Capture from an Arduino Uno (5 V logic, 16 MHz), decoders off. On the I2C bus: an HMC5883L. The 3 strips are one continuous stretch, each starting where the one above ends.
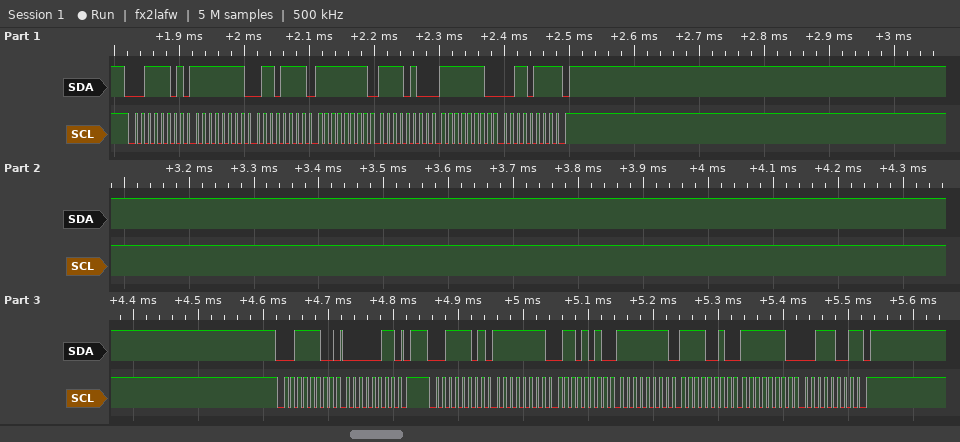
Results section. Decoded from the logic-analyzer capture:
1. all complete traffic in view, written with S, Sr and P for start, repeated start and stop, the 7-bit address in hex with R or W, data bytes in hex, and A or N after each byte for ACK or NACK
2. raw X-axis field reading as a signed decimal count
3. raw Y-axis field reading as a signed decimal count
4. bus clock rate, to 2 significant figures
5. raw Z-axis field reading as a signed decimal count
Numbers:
S 1ER A FF A 6F A FF A F4 A FE A 37 N P S 1EW A 03 A P S 1ER A FF A 6A A FF A F2 A FE A 39 N P
-150
-455
100 kHz
-14
